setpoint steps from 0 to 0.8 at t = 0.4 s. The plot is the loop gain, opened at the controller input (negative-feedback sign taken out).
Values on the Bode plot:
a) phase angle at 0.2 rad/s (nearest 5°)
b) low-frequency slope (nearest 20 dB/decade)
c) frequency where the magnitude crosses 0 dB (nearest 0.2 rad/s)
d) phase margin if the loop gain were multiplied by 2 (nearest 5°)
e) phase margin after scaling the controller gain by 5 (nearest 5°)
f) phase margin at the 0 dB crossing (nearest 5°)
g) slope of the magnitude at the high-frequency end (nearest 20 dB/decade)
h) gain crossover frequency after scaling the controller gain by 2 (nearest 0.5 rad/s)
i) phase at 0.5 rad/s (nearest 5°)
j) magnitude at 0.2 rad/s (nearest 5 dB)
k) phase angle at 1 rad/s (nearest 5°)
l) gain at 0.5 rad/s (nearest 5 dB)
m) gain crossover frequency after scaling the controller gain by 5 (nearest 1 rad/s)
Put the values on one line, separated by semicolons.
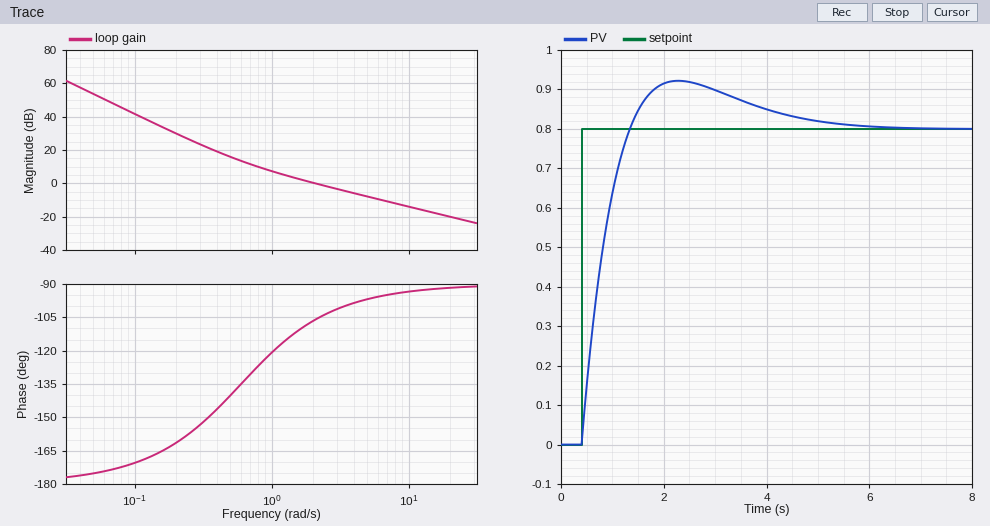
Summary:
-160°; -40 dB/decade; 2.0 rad/s; 80°; 85°; 75°; -20 dB/decade; 4.0 rad/s; -140°; 30 dB; -120°; 15 dB; 10 rad/s
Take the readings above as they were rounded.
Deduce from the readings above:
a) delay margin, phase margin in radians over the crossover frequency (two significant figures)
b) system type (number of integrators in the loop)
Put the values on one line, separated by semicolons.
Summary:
0.65 s; 2
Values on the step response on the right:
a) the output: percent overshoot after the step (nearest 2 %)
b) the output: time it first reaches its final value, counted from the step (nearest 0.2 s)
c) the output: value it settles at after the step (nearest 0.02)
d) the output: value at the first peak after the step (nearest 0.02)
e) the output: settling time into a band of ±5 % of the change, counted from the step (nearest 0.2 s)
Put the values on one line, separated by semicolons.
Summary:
16 %; 1.0 s; 0.80; 0.92; 3.8 s
